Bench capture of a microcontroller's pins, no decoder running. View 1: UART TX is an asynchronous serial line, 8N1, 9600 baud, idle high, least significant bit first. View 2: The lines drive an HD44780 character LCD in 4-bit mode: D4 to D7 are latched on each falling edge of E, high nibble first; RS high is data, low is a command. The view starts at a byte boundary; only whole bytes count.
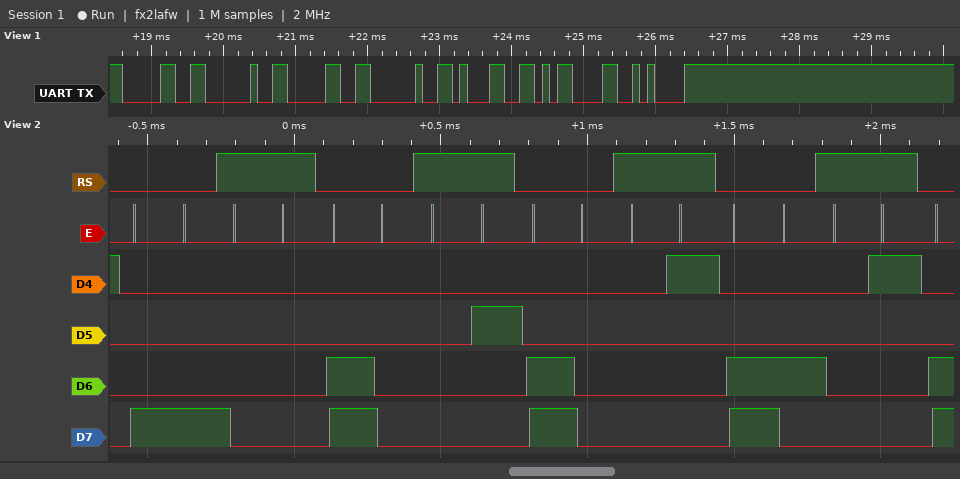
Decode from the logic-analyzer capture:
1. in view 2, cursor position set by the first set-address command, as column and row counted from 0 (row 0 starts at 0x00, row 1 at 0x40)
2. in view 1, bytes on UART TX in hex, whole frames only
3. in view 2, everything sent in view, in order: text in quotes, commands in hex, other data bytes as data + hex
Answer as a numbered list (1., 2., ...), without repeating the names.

1. column 8, row 0
2. 30 20 30 20 31 0D 0A
3. 0x88 data 00 0xC0 data 02 0xC0 data 01 0xC4 data 01
